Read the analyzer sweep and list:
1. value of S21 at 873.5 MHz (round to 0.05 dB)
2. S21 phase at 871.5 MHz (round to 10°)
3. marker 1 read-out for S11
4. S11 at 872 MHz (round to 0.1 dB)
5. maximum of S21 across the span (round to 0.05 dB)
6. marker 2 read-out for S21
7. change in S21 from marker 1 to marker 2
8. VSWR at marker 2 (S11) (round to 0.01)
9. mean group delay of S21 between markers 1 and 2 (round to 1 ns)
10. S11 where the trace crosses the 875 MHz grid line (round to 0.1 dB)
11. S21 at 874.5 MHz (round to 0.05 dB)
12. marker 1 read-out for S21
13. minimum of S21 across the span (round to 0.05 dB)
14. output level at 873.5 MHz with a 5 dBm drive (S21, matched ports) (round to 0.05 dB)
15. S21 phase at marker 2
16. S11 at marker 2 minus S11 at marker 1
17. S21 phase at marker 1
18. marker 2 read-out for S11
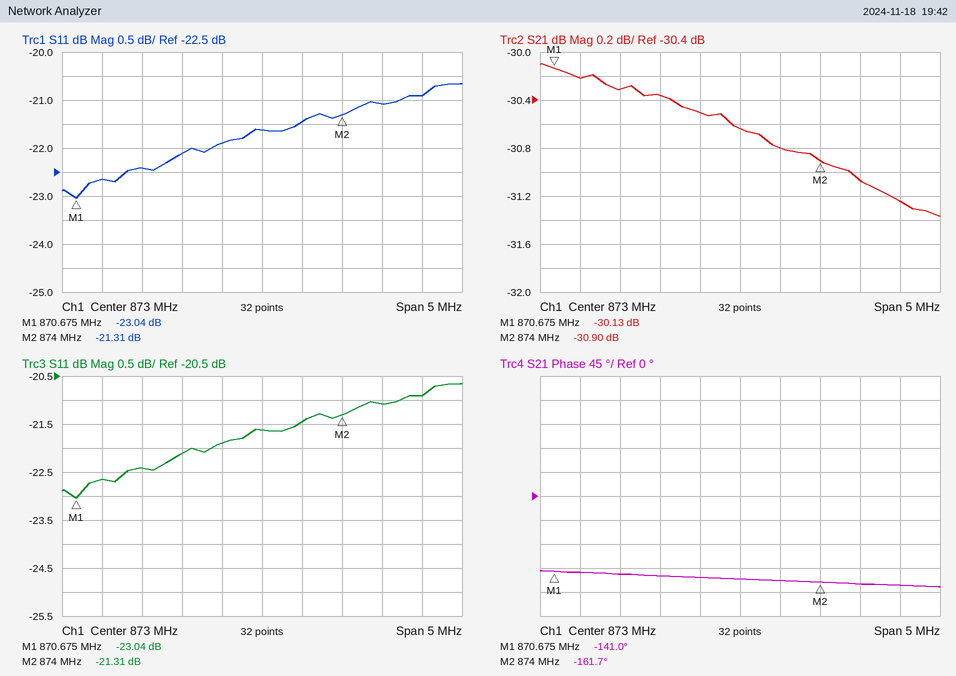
-30.80 dB
-150°
-23.04 dB
-22.1 dB
-30.10 dB
-30.90 dB
-0.77 dB
1.19
17 ns
-20.9 dB
-31.05 dB
-30.13 dB
-31.35 dB
-25.80 dBm
-161.7°
1.73 dB
-141.0°
-21.31 dB
